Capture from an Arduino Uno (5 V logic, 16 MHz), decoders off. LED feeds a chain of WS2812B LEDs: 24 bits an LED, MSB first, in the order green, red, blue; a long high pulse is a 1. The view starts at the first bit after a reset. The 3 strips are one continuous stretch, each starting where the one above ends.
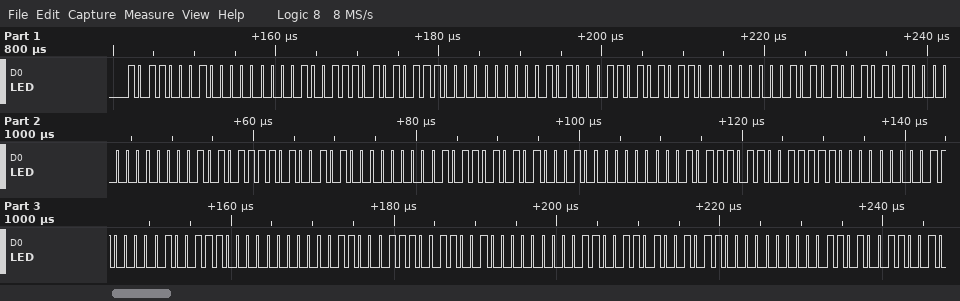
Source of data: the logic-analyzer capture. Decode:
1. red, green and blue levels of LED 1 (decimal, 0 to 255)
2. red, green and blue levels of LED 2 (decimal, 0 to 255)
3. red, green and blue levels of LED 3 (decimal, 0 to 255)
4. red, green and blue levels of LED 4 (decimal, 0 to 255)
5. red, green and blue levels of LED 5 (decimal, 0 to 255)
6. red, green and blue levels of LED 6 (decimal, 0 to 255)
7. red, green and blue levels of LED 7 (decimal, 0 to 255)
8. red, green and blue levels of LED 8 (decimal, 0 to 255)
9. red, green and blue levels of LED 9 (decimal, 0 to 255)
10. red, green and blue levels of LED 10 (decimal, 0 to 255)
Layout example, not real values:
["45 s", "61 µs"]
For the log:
["0, 177, 78", "0, 174, 81", "0, 171, 84", "0, 168, 87", "0, 165, 90", "0, 162, 93", "0, 159, 96", "0, 156, 99", "0, 153, 102", "0, 150, 105"]
